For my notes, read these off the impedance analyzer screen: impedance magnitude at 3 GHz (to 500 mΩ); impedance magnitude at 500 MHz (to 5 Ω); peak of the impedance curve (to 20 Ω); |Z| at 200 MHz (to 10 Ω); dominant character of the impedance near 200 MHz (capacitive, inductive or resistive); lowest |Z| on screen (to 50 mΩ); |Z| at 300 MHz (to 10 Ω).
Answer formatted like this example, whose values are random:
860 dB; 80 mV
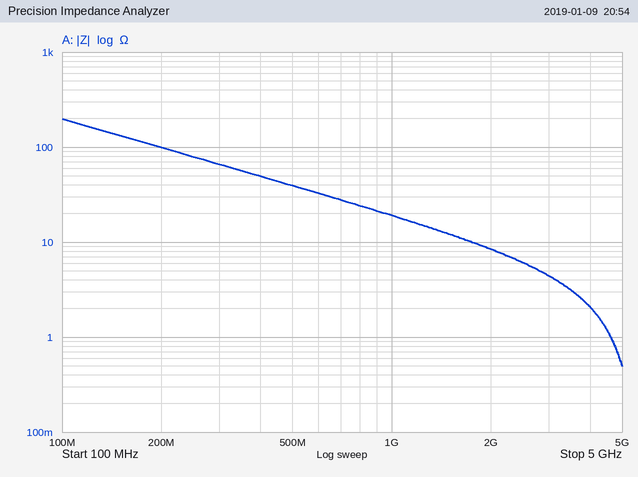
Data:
4.5 Ω; 40 Ω; 200 Ω; 100 Ω; capacitive; 500 mΩ; 70 Ω
